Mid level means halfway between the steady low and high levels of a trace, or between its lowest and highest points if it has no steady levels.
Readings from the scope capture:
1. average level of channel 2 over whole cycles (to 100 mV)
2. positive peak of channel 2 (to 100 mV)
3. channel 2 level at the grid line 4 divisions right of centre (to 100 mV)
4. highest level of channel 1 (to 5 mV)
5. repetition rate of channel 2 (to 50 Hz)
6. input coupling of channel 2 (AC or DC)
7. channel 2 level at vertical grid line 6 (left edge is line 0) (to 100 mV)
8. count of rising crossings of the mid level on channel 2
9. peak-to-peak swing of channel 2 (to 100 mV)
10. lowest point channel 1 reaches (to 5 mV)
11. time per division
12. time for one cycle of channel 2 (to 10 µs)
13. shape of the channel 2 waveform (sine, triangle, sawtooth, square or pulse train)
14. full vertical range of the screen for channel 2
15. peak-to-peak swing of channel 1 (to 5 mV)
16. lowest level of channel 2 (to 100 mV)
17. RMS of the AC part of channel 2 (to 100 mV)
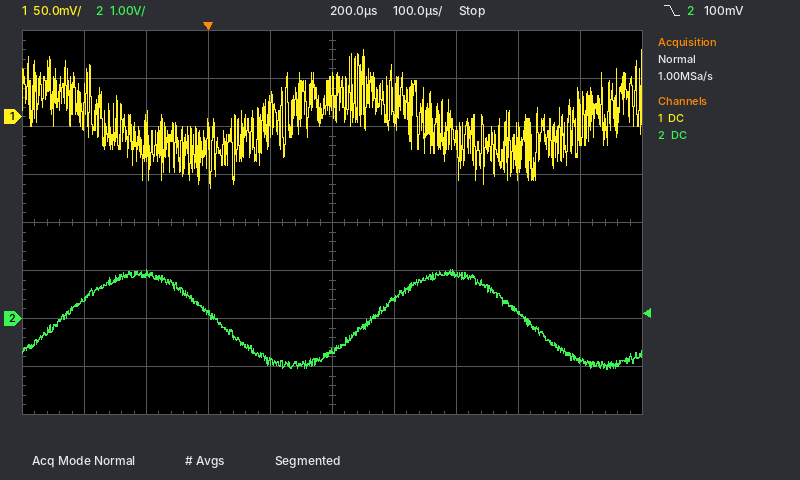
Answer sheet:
0.0 V
1.0 V
-900 mV
70 mV
2.00 kHz
DC
400 mV
2
2.1 V
-75 mV
100 µs
500 µs
sine
8 V
145 mV
-1.1 V
700 mV
